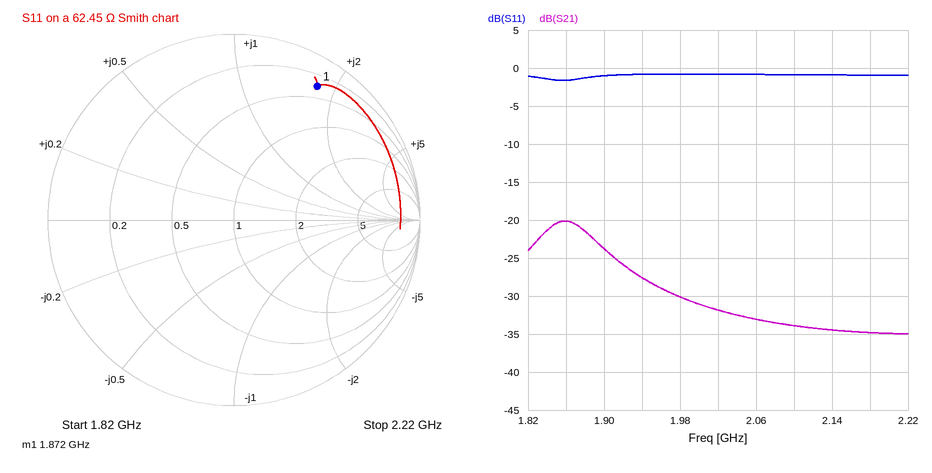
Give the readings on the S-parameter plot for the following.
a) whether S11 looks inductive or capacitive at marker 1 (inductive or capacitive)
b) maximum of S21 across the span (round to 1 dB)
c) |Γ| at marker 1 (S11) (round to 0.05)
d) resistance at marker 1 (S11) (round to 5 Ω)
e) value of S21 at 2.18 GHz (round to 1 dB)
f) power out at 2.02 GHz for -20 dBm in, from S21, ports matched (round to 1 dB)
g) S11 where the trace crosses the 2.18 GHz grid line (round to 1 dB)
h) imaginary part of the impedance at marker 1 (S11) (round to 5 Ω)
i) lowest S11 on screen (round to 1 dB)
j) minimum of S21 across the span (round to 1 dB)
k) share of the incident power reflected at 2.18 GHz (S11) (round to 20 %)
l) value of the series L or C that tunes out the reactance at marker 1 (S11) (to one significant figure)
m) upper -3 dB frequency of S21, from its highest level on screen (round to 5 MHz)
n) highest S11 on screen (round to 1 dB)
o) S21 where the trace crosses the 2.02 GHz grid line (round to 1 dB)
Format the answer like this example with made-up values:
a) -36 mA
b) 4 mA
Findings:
a) inductive
b) -20 dB
c) 0.85
d) 20 Ω
e) -35 dB
f) -52 dBm
g) -1 dB
h) +110 Ω
i) -2 dB
j) -35 dB
k) 80 %
l) 800 fF
m) 1.895 GHz
n) -1 dB
o) -32 dB
